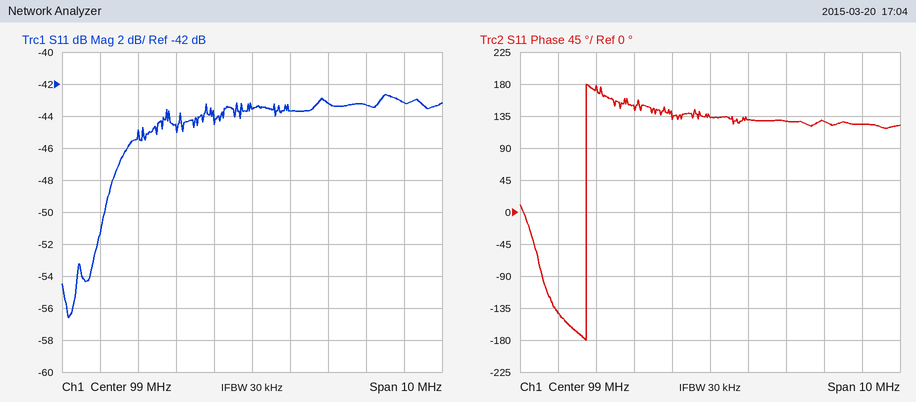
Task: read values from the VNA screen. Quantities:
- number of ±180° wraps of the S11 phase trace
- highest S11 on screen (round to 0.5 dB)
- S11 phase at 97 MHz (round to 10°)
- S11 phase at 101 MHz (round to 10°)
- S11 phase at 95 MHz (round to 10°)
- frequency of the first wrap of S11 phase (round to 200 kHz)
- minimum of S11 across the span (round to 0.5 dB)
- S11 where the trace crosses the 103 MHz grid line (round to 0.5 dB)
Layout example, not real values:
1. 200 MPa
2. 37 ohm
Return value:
1. 1
2. -42.5 dB
3. 150°
4. 130°
5. -140°
6. 95.8 MHz
7. -56.5 dB
8. -43.0 dB
